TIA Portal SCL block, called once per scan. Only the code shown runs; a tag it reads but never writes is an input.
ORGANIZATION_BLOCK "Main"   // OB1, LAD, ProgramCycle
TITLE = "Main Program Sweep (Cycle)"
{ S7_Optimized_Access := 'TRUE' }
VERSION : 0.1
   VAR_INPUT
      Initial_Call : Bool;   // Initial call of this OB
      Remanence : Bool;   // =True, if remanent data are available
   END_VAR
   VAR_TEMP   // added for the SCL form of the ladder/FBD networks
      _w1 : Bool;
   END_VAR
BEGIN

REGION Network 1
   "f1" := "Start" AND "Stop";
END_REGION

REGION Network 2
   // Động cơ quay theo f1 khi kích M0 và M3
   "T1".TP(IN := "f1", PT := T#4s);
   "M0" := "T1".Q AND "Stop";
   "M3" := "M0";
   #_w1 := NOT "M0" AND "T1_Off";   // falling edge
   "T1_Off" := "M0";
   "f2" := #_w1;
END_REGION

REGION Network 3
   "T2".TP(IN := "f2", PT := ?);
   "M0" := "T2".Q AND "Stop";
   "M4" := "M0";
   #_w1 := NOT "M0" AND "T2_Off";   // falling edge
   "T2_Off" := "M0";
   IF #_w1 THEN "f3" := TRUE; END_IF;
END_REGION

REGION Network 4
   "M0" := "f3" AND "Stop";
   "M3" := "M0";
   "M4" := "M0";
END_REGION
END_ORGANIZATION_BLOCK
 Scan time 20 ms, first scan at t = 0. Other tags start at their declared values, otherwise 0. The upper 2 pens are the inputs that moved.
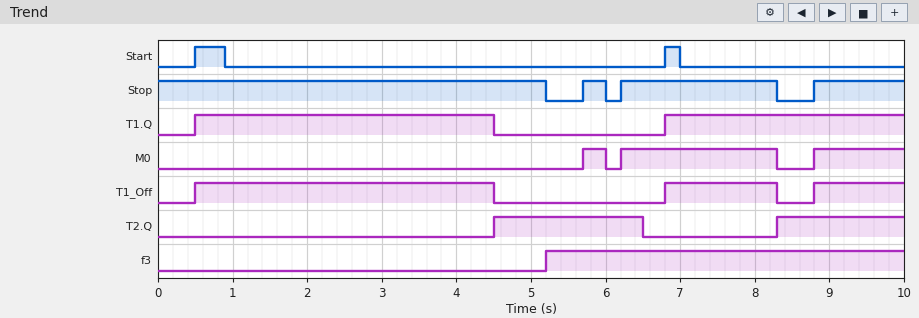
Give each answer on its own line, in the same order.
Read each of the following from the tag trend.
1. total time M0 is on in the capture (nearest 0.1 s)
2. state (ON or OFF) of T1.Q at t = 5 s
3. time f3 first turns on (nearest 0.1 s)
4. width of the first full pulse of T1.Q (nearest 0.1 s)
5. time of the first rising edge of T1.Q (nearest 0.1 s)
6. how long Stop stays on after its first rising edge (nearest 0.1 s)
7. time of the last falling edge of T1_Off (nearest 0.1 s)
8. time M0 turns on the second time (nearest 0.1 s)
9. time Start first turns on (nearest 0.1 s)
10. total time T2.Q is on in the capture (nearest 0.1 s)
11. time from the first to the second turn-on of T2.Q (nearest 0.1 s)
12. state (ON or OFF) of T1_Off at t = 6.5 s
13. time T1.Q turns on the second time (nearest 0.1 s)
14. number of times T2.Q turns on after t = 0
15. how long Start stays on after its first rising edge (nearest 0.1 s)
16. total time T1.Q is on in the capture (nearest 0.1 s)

3.6 s
OFF
5.2 s
4.0 s
0.5 s
0.3 s
8.3 s
6.2 s
0.5 s
3.7 s
3.8 s
OFF
6.8 s
2
0.4 s
7.2 s
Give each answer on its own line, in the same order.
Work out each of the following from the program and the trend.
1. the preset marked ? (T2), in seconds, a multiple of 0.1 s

2.0 s
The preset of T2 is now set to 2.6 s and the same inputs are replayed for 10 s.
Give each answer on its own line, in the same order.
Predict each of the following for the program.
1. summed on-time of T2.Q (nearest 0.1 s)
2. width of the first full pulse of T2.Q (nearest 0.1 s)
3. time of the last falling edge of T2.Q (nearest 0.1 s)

4.3 s
2.6 s
7.1 s
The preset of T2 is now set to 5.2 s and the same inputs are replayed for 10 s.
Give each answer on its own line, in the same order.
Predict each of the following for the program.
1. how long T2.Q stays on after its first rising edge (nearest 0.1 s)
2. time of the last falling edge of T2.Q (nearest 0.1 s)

5.2 s
9.7 s
